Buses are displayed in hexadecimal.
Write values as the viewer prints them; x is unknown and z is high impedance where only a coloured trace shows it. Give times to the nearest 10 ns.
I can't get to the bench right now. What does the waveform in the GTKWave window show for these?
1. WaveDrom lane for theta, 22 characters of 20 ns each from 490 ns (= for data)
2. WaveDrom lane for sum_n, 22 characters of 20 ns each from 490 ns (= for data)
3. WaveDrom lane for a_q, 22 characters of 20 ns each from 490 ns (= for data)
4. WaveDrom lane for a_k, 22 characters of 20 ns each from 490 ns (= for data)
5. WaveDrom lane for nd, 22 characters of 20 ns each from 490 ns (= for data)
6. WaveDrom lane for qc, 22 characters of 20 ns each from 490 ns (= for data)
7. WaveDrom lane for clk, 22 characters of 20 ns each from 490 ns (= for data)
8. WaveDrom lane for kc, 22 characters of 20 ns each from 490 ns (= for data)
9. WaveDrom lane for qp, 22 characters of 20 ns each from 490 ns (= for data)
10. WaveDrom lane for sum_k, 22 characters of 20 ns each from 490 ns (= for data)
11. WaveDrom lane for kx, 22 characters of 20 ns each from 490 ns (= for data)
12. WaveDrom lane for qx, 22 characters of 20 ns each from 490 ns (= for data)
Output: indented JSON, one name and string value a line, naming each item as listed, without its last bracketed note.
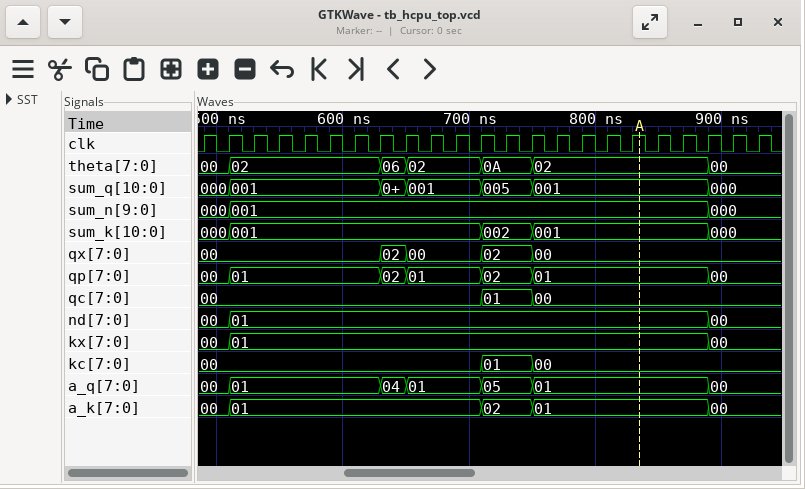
{
  "WaveDrom lane for theta, 22 characters of 20 ns each from 490 ns": "{name: 'theta', wave: '==.....==..=.=......=.', data: '00 02 06 02 0A 02 00'}",
  "WaveDrom lane for sum_n, 22 characters of 20 ns each from 490 ns": "{name: 'sum_n', wave: '==..................=.', data: '000 001 000'}",
  "WaveDrom lane for a_q, 22 characters of 20 ns each from 490 ns": "{name: 'a_q', wave: '==.....==..=.=......=.', data: '00 01 04 01 05 01 00'}",
  "WaveDrom lane for a_k, 22 characters of 20 ns each from 490 ns": "{name: 'a_k', wave: '==.........=.=......=.', data: '00 01 02 01 00'}",
  "WaveDrom lane for nd, 22 characters of 20 ns each from 490 ns": "{name: 'nd', wave: '==..................=.', data: '00 01 00'}",
  "WaveDrom lane for qc, 22 characters of 20 ns each from 490 ns": "{name: 'qc', wave: '=..........=.=........', data: '00 01 00'}",
  "WaveDrom lane for clk, 22 characters of 20 ns each from 490 ns": "{name: 'clk', wave: 'p.....................'}",
  "WaveDrom lane for kc, 22 characters of 20 ns each from 490 ns": "{name: 'kc', wave: '=..........=.=........', data: '00 01 00'}",
  "WaveDrom lane for qp, 22 characters of 20 ns each from 490 ns": "{name: 'qp', wave: '==.....==..=.=......=.', data: '00 01 02 01 02 01 00'}",
  "WaveDrom lane for sum_k, 22 characters of 20 ns each from 490 ns": "{name: 'sum_k', wave: '==.........=.=......=.', data: '000 001 002 001 000'}",
  "WaveDrom lane for kx, 22 characters of 20 ns each from 490 ns": "{name: 'kx', wave: '==..................=.', data: '00 01 00'}",
  "WaveDrom lane for qx, 22 characters of 20 ns each from 490 ns": "{name: 'qx', wave: '=......==..=.=........', data: '00 02 00 02 00'}"
}
